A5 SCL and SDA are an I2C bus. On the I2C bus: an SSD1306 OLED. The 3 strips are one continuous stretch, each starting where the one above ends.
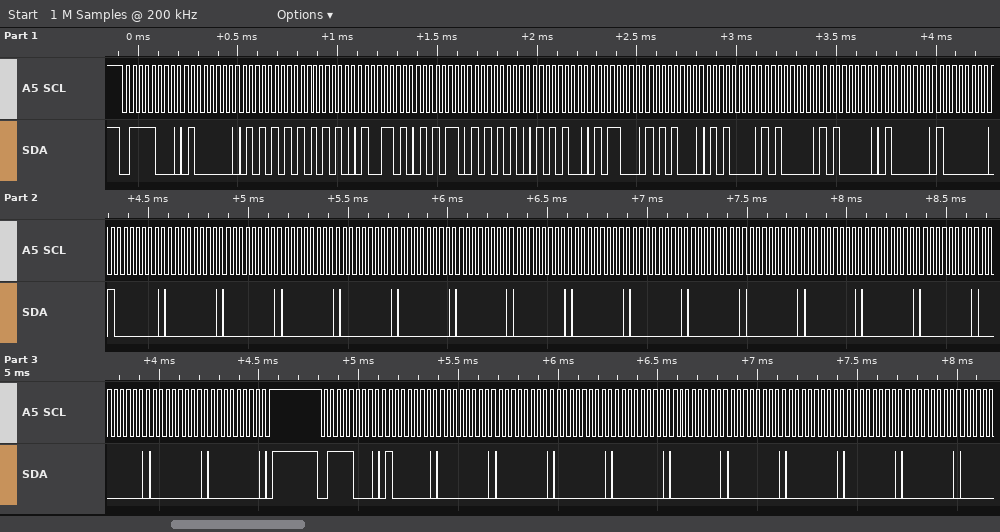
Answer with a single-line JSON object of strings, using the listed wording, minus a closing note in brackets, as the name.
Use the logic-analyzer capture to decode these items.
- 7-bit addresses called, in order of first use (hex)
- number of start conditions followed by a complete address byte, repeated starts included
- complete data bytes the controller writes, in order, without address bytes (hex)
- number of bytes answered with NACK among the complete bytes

{"7-bit addresses called, in order of first use": "0x3C", "number of start conditions followed by a complete address byte, repeated starts included": "2", "complete data bytes the controller writes, in order, without address bytes": "40 55 AA 4D 56 AA 54 58 A8 50 A0 A0 40 80 80 00 00 00 00 00 00 00 00 00 00 00 00 00 00 00 00 00 40 00 00 00 00 00 00 00 00 00", "number of bytes answered with NACK among the complete bytes": "0"}
